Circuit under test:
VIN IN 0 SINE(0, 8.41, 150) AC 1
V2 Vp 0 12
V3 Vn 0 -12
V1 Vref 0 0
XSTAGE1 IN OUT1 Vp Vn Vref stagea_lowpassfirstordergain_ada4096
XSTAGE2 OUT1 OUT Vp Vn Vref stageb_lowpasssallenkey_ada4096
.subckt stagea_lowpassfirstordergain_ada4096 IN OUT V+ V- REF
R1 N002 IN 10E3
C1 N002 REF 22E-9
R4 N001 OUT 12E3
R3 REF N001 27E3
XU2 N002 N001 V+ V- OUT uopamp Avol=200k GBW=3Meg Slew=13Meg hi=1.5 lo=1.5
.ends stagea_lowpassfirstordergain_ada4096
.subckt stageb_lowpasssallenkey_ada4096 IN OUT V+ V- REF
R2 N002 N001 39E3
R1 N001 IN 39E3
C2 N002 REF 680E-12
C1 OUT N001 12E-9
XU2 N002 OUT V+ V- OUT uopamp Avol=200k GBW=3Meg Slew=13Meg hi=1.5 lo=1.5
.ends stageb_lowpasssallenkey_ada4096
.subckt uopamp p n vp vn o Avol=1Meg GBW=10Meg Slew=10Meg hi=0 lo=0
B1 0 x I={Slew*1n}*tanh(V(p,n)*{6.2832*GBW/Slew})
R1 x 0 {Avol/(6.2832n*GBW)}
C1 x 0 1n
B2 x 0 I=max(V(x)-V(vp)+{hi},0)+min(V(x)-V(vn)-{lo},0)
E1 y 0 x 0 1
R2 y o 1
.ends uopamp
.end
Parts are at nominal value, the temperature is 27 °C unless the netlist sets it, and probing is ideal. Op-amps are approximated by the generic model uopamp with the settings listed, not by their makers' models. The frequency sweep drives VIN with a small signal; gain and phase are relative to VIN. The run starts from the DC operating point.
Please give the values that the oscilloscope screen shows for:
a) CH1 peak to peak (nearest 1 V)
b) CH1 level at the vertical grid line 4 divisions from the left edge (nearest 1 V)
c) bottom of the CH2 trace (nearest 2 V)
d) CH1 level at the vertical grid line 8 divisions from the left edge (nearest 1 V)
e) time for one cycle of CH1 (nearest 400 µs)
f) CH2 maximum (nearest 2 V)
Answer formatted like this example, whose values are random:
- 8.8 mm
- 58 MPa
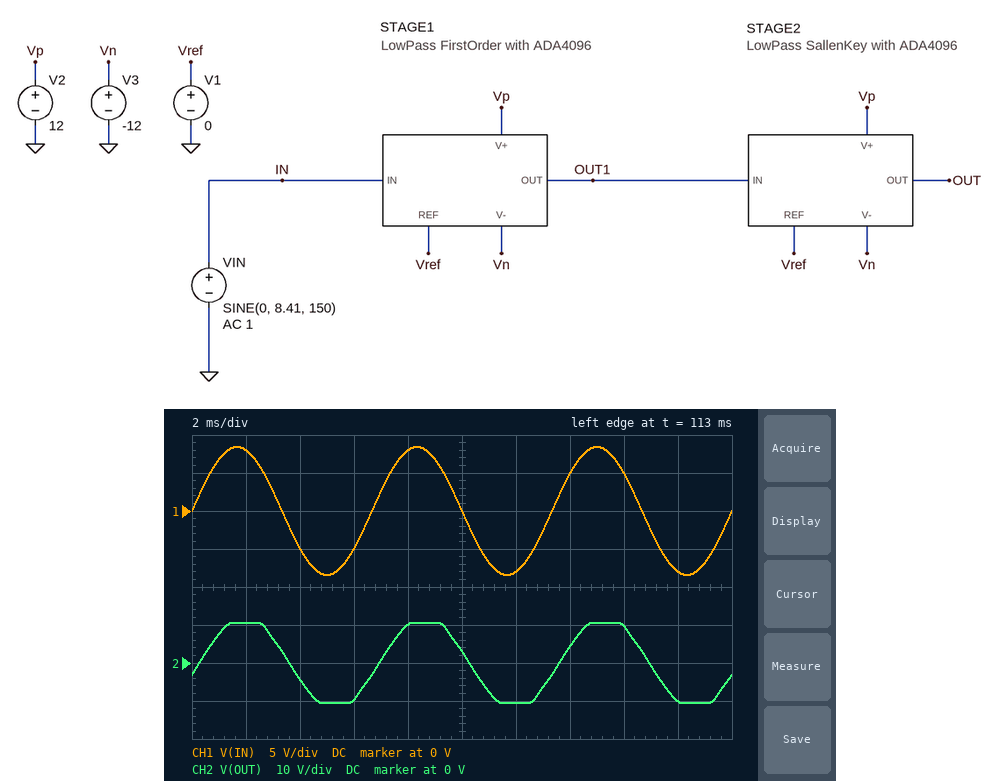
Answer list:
- 17 V
- 8 V
- -10 V
- 5 V
- 6.8 ms
- 10 V
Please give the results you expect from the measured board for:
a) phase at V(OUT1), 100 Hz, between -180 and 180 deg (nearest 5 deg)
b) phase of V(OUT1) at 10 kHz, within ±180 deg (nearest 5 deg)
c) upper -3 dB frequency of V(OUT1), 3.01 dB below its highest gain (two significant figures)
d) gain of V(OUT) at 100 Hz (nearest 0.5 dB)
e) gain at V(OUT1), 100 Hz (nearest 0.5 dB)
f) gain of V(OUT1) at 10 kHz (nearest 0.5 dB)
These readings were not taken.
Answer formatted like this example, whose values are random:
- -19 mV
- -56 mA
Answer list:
- -10 deg
- -85 deg
- 720 Hz
- 3.0 dB
- 3.0 dB
- -19.5 dB
